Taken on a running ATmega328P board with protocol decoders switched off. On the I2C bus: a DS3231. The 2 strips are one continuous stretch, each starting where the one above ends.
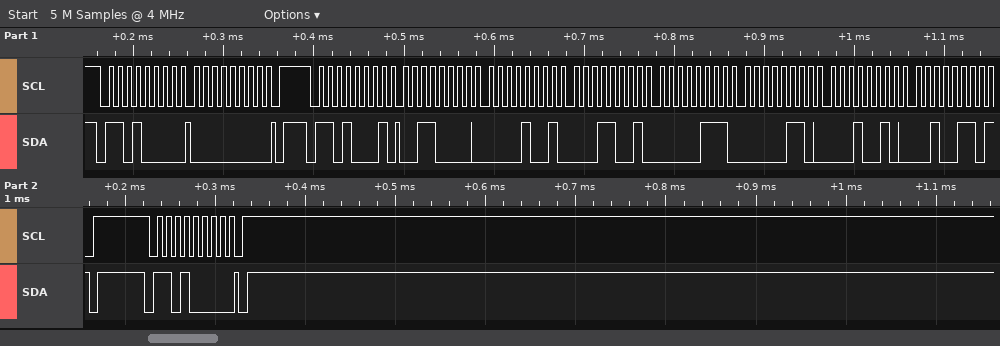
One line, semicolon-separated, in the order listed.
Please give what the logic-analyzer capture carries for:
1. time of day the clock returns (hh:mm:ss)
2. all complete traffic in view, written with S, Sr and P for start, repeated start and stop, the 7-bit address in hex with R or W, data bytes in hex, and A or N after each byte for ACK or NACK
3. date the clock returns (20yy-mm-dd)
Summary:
19:09:30; S 68W A 00 A P S 68R A 30 A 09 A 19 A 07 A 06 A 12 A 26 N P S 68W A P; 2026-12-06
